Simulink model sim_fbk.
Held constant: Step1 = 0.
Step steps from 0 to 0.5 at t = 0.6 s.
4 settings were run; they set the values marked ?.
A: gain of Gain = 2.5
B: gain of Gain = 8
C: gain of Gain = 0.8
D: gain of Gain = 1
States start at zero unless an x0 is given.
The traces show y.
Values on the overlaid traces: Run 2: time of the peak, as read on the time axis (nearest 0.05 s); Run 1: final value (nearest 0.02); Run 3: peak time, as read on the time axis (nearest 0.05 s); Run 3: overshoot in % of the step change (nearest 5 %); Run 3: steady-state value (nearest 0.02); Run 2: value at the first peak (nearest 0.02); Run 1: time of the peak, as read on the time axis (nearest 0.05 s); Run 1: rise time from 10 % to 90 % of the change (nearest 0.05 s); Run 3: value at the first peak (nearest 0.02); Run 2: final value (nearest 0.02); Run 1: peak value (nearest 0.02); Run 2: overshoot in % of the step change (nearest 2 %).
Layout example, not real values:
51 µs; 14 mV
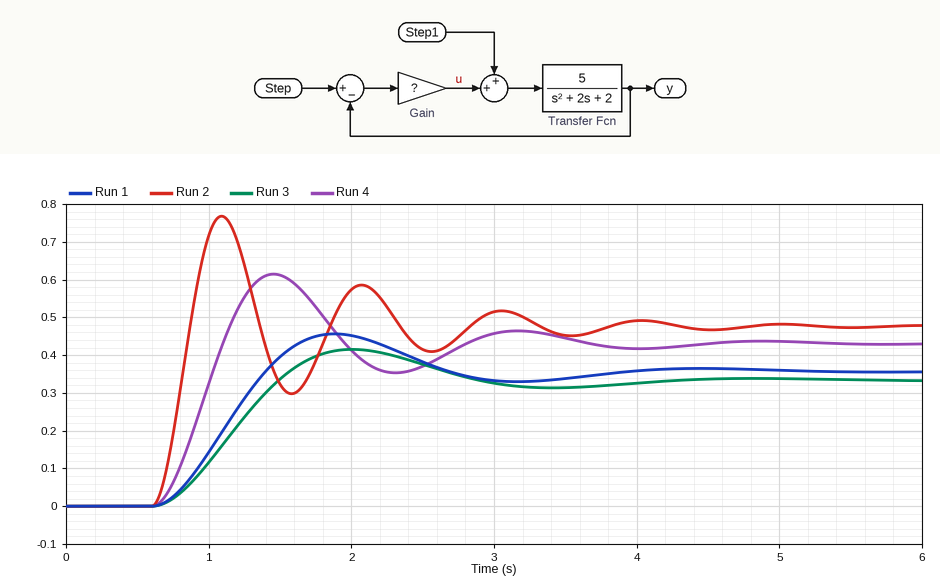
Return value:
1.10 s; 0.36; 2.00 s; 25 %; 0.34; 0.76; 1.90 s; 0.55 s; 0.42; 0.48; 0.46; 62 %
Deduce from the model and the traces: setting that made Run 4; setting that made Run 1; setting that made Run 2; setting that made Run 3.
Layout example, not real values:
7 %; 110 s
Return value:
A; D; B; C
